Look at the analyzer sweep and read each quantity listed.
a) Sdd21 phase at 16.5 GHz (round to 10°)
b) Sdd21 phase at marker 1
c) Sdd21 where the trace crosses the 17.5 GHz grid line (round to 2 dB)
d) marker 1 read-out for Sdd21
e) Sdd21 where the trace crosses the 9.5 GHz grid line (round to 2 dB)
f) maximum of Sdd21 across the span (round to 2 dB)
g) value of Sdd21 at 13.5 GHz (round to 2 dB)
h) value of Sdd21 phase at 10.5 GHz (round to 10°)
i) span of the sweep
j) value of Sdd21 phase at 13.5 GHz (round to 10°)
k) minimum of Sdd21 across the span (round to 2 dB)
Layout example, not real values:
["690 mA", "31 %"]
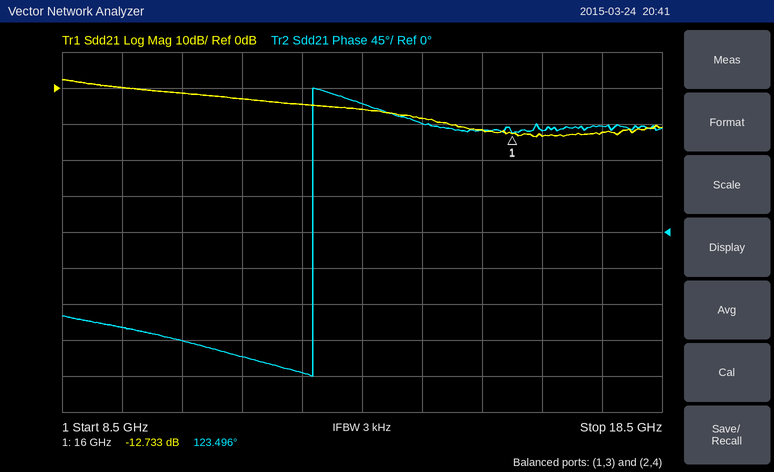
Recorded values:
["130°", "123.496°", "-12 dB", "-12.733 dB", "0 dB", "2 dB", "-6 dB", "-140°", "10 GHz", "160°", "-14 dB"]
